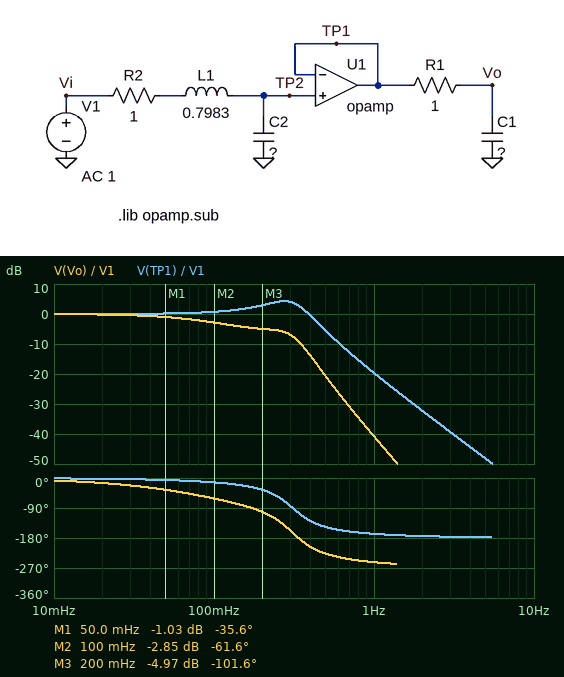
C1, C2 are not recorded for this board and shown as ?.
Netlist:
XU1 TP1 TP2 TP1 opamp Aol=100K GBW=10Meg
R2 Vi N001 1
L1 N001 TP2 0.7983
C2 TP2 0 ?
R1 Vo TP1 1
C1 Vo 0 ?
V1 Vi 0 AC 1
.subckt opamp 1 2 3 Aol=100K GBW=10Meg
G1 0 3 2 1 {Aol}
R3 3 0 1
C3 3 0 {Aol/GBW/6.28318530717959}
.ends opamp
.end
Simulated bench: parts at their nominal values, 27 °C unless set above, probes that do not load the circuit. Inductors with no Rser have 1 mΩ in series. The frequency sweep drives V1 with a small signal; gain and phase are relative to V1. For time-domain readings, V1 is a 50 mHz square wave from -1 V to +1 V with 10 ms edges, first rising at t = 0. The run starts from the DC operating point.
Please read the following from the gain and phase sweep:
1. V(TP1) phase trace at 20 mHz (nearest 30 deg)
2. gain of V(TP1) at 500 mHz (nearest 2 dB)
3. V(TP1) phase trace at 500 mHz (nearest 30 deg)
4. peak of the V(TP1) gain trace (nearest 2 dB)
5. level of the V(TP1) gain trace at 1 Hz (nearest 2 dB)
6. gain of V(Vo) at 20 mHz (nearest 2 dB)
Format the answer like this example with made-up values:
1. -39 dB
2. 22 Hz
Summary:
1. 0 deg
2. -6 dB
3. -150 deg
4. 4 dB
5. -20 dB
6. 0 dB
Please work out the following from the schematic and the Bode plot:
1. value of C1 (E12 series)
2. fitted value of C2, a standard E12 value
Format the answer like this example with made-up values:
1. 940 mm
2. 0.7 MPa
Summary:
1. 1.8 F
2. 330 mF
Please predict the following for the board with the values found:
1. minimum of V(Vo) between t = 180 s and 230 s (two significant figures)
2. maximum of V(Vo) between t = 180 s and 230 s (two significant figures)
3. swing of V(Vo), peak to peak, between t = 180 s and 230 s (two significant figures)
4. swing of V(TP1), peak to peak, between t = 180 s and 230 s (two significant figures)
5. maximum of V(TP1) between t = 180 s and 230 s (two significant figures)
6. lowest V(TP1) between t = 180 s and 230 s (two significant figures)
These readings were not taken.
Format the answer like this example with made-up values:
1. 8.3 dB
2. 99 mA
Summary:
1. -990 mV
2. 990 mV
3. 2.0 V
4. 3.4 V
5. 1.7 V
6. -1.7 V
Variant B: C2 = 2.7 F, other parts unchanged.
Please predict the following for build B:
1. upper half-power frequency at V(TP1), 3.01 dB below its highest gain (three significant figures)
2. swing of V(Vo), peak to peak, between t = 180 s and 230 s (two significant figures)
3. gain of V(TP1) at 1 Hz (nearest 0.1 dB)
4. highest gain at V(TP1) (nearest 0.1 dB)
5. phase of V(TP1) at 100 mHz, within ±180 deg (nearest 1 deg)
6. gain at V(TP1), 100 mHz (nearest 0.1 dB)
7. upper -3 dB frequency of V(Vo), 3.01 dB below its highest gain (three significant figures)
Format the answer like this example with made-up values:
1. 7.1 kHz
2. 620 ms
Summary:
1. 78.4 mHz
2. 1.9 V
3. -38.7 dB
4. 0 dB
5. -85 deg
6. -4.6 dB
7. 55.6 mHz
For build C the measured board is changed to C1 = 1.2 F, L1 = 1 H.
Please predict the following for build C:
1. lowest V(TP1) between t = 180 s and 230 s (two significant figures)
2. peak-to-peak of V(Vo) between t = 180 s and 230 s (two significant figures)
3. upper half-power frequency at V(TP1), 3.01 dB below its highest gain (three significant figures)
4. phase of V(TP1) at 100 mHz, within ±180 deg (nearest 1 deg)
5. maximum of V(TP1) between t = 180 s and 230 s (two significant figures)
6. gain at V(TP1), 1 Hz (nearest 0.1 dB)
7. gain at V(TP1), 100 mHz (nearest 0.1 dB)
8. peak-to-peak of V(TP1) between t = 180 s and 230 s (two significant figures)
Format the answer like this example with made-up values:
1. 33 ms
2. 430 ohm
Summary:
1. -1.8 V
2. 2.1 V
3. 326 mHz
4. -13 deg
5. 1.8 V
6. -21.7 dB
7. 1.0 dB
8. 3.6 V
